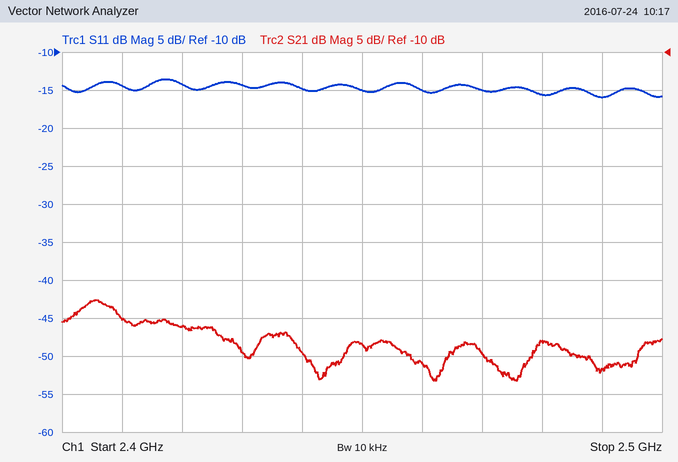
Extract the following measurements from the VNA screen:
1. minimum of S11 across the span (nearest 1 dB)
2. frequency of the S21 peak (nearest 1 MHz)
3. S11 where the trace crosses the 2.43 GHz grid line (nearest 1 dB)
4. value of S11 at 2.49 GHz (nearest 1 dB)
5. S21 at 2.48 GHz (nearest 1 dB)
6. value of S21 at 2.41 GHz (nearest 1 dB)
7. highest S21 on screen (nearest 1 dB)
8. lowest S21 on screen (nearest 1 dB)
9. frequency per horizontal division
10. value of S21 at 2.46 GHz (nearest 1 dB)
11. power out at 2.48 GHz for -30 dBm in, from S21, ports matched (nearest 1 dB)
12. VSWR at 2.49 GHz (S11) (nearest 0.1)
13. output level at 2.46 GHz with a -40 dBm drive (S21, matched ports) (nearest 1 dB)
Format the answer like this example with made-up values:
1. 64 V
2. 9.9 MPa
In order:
1. -16 dB
2. 2.406 GHz
3. -14 dB
4. -16 dB
5. -48 dB
6. -45 dB
7. -43 dB
8. -53 dB
9. 10 MHz
10. -51 dB
11. -78 dBm
12. 1.4
13. -91 dBm
